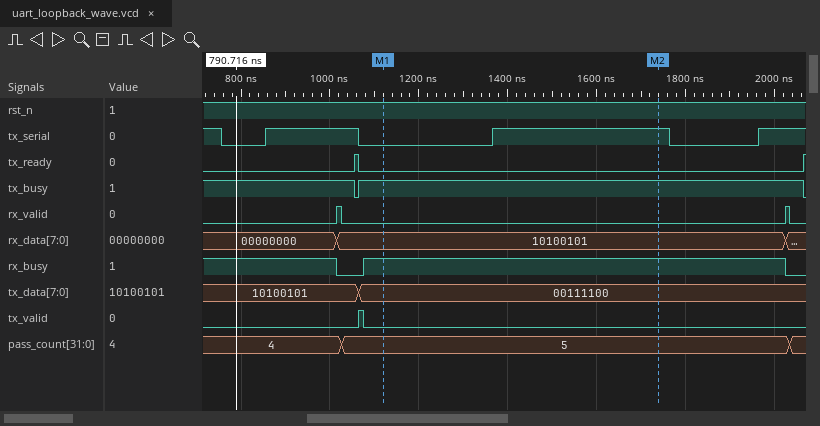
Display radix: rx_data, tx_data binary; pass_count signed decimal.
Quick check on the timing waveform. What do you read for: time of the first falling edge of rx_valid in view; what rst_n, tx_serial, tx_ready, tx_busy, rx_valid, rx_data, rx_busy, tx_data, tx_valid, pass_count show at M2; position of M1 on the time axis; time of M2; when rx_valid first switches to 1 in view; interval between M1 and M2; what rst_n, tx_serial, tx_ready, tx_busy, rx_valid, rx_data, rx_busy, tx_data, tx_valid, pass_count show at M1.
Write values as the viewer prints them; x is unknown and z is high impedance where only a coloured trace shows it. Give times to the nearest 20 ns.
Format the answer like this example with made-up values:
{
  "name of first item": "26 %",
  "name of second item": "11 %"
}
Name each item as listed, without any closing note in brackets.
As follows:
{
  "time of the first falling edge of rx_valid in view": "1020 ns",
  "what rst_n, tx_serial, tx_ready, tx_busy, rx_valid, rx_data, rx_busy, tx_data, tx_valid, pass_count show at M2": "rst_n=1, tx_serial=1, tx_ready=0, tx_busy=1, rx_valid=0, rx_data=10100101, rx_busy=1, tx_data=00111100, tx_valid=0, pass_count=5",
  "position of M1 on the time axis": "1120 ns",
  "time of M2": "1740 ns",
  "when rx_valid first switches to 1 in view": "1020 ns",
  "interval between M1 and M2": "620 ns",
  "what rst_n, tx_serial, tx_ready, tx_busy, rx_valid, rx_data, rx_busy, tx_data, tx_valid, pass_count show at M1": "rst_n=1, tx_serial=0, tx_ready=0, tx_busy=1, rx_valid=0, rx_data=10100101, rx_busy=1, tx_data=00111100, tx_valid=0, pass_count=5"
}
